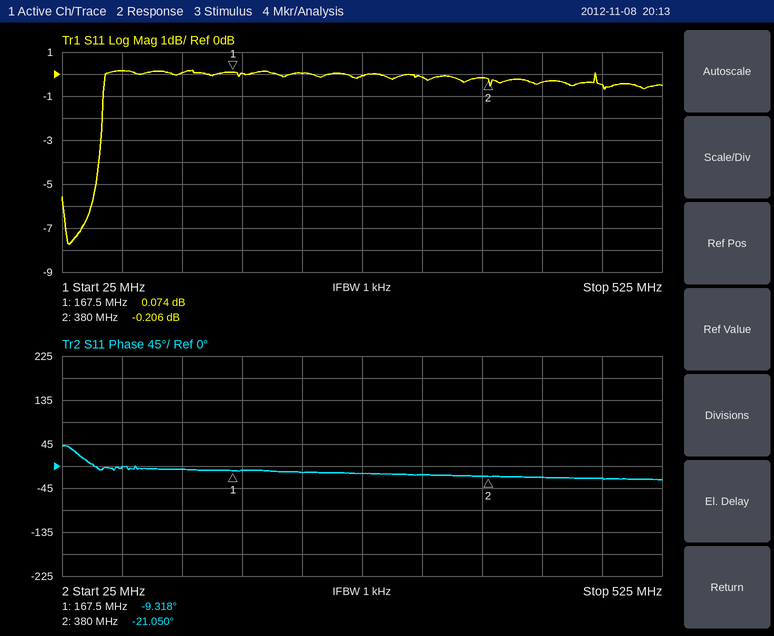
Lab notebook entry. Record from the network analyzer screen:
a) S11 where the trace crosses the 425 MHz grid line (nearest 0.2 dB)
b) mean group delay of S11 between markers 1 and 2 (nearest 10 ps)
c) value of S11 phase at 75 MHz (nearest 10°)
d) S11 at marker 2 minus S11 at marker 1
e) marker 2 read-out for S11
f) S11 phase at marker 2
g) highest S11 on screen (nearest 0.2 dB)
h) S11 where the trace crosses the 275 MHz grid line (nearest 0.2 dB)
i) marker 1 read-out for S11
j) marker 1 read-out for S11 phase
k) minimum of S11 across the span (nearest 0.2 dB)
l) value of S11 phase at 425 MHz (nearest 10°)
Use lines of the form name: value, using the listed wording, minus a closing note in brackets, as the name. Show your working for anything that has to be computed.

S11 where the trace crosses the 425 MHz grid line: -0.4 dB
mean group delay of S11 between markers 1 and 2: −(-21.05° − (-9.318°))/(360° × 212.5 MHz) ≈ 153 ps, so 150 ps to the nearest 10 ps
value of S11 phase at 75 MHz: 0°
S11 at marker 2 minus S11 at marker 1: -0.206 − (0.074) = -0.280 dB
marker 2 read-out for S11: -0.206 dB
S11 phase at marker 2: -21.050°
highest S11 on screen: 0.2 dB
S11 where the trace crosses the 275 MHz grid line: 0.0 dB
marker 1 read-out for S11: 0.074 dB
marker 1 read-out for S11 phase: -9.318°
minimum of S11 across the span: -7.8 dB
value of S11 phase at 425 MHz: -20°
